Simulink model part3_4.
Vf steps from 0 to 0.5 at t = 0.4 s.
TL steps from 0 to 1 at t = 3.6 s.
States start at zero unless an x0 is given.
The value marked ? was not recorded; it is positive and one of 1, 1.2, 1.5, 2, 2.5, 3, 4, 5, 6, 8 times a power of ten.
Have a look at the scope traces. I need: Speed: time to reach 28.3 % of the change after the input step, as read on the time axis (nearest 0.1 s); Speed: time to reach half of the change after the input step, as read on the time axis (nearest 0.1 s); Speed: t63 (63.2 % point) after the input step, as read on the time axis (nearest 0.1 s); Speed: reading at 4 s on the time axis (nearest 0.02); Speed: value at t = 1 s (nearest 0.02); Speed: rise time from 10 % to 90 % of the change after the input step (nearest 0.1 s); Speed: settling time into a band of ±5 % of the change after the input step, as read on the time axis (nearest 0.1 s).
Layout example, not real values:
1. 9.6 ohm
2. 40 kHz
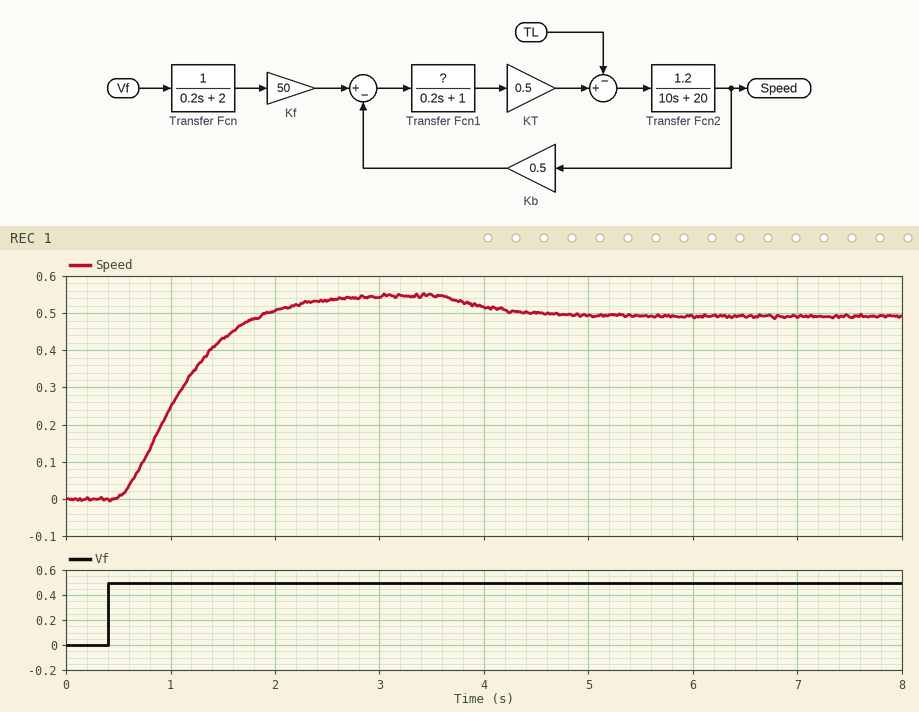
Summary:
1. 0.8 s
2. 1.1 s
3. 1.2 s
4. 0.52
5. 0.24
6. 1.2 s
7. 2.2 s
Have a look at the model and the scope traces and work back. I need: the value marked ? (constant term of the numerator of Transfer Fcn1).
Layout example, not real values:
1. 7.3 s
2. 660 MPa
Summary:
1. 1.5
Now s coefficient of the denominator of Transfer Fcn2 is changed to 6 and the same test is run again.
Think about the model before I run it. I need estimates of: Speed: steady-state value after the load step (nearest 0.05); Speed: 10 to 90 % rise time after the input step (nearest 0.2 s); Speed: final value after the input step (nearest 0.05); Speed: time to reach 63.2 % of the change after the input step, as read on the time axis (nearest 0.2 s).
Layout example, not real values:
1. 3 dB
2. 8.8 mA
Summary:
1. 0.50
2. 0.8 s
3. 0.55
4. 1.0 s
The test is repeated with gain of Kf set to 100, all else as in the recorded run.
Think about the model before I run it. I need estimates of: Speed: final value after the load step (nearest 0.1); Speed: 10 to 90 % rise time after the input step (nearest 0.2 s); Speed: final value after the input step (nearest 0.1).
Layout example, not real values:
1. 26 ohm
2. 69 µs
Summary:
1. 1.0
2. 1.2 s
3. 1.1
